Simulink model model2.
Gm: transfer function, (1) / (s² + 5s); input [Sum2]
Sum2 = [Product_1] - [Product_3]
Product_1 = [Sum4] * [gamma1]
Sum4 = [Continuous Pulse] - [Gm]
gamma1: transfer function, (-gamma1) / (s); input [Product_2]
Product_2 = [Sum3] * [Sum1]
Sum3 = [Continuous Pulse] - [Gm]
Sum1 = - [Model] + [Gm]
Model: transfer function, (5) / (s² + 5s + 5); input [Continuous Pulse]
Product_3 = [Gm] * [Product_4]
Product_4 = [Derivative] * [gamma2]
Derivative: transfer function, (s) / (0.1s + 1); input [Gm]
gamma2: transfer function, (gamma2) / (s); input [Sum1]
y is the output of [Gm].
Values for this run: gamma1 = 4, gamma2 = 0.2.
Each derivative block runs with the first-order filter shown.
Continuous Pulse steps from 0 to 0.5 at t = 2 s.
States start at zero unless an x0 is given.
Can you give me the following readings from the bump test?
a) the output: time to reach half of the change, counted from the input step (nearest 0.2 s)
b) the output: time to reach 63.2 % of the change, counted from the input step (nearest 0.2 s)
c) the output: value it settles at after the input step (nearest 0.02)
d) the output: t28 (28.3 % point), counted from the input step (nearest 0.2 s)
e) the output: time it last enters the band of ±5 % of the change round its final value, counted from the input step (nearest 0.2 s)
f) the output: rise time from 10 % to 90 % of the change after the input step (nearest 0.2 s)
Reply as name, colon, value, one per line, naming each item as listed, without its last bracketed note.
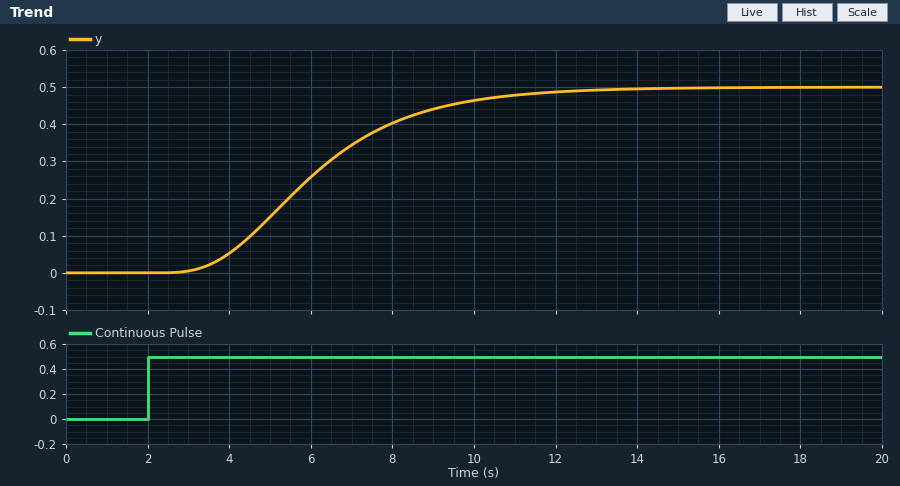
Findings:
the output: time to reach half of the change, counted from the input step: 4.0 s
the output: time to reach 63.2 % of the change, counted from the input step: 4.6 s
the output: value it settles at after the input step: 0.50
the output: t28 (28.3 % point), counted from the input step: 3.0 s
the output: time it last enters the band of ±5 % of the change round its final value, counted from the input step: 8.8 s
the output: rise time from 10 % to 90 % of the change after the input step: 5.4 s
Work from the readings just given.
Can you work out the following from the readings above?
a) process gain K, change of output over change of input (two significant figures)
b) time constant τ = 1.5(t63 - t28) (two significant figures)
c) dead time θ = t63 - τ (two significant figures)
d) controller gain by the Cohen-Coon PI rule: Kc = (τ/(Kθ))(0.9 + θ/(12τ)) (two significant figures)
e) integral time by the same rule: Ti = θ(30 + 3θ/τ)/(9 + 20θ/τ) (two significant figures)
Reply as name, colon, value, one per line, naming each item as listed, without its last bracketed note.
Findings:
process gain K, change of output over change of input: 1.0
time constant τ = 1.5(t63 - t28): 2.4 s
dead time θ = t63 - τ: 2.2 s
controller gain by the Cohen-Coon PI rule: Kc = (τ/(Kθ))(0.9 + θ/(12τ)): 1.1
integral time by the same rule: Ti = θ(30 + 3θ/τ)/(9 + 20θ/τ): 2.6 s
